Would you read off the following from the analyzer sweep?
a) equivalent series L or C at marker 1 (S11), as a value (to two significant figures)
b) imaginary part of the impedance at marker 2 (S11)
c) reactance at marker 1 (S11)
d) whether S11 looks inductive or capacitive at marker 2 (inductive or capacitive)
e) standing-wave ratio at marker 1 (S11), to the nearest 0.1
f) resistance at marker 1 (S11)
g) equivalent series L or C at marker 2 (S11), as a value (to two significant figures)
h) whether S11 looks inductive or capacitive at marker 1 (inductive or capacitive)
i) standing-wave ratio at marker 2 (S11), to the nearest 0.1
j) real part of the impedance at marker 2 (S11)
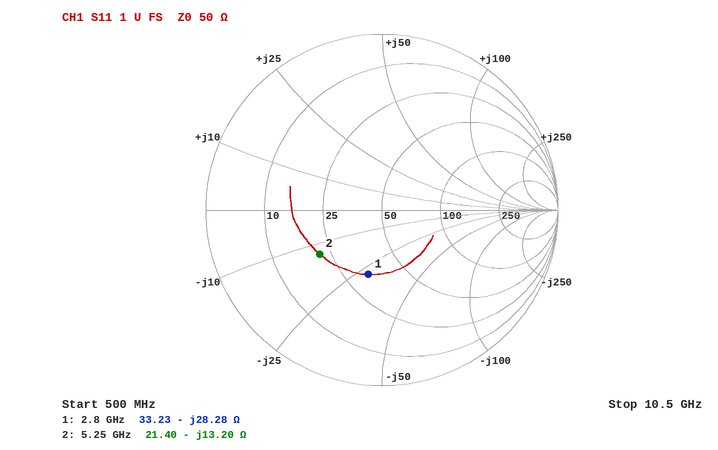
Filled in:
2.0 pF
-13.20 Ω
-28.28 Ω
capacitive
2.2
33.23 Ω
2.3 pF
capacitive
2.5
21.40 Ω
